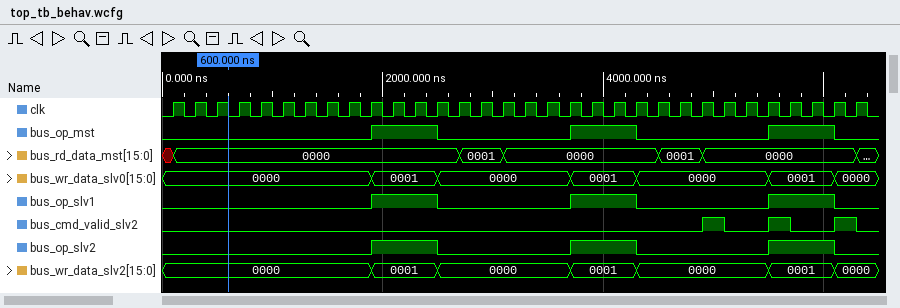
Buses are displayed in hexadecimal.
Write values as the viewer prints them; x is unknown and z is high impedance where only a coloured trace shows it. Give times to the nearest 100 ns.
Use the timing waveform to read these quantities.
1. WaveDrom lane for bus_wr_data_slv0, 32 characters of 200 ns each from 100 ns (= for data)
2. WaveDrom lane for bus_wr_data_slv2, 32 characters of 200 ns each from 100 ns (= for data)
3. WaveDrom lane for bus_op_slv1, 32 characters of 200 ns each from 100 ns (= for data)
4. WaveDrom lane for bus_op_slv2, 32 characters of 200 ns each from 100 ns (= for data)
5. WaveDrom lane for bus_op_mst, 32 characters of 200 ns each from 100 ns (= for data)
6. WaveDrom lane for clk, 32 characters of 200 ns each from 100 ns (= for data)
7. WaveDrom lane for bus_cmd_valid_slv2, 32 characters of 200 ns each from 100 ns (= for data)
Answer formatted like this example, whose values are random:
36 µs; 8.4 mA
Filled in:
{name: 'bus_wr_data_slv0', wave: '=........=..=.....=..=.....=..=.', data: '0000 0001 0000 0001 0000 0001 0000'}; {name: 'bus_wr_data_slv2', wave: '=........=..=.....=..=.....=..=.', data: '0000 0001 0000 0001 0000 0001 0000'}; {name: 'bus_op_slv1', wave: '0........1..0.....1..0.....1..0.'}; {name: 'bus_op_slv2', wave: '0........1..0.....1..0.....1..0.'}; {name: 'bus_op_mst', wave: '0........1..0.....1..0.....1..0.'}; {name: 'clk', wave: 'p...............................'}; {name: 'bus_cmd_valid_slv2', wave: '0.......................10.10.10'}
